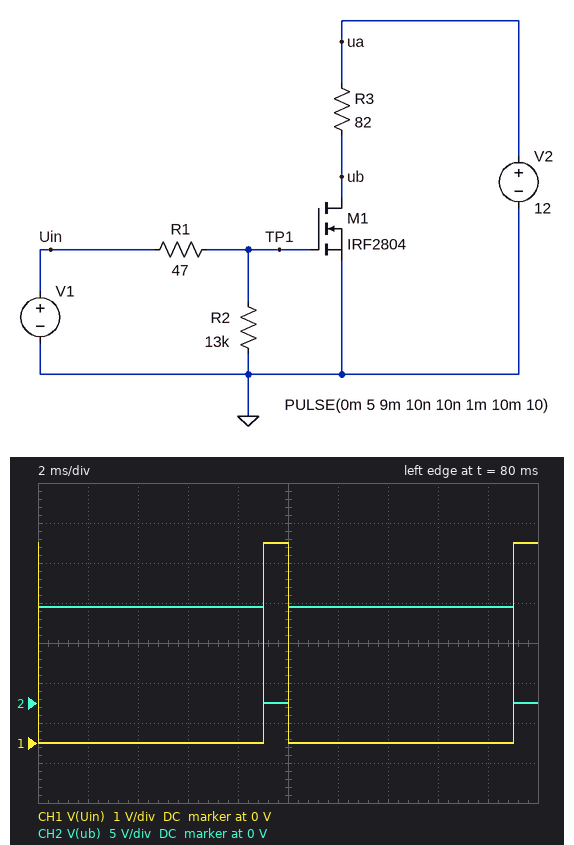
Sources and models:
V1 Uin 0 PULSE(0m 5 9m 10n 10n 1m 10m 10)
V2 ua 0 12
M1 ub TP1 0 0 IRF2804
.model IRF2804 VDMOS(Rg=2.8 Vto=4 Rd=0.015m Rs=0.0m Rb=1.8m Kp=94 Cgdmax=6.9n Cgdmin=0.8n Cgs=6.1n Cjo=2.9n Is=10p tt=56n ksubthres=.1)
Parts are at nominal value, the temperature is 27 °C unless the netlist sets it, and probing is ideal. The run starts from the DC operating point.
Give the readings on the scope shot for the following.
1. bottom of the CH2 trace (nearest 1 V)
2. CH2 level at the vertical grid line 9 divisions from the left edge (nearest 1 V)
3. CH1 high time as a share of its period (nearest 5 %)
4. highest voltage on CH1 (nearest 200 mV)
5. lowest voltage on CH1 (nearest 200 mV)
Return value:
0 V
12 V
10 %
5.0 V
0 V
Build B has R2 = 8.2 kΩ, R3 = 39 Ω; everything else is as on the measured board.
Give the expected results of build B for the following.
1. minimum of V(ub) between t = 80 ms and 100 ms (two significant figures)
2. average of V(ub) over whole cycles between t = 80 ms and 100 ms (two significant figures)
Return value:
2.9 mV
11 V
